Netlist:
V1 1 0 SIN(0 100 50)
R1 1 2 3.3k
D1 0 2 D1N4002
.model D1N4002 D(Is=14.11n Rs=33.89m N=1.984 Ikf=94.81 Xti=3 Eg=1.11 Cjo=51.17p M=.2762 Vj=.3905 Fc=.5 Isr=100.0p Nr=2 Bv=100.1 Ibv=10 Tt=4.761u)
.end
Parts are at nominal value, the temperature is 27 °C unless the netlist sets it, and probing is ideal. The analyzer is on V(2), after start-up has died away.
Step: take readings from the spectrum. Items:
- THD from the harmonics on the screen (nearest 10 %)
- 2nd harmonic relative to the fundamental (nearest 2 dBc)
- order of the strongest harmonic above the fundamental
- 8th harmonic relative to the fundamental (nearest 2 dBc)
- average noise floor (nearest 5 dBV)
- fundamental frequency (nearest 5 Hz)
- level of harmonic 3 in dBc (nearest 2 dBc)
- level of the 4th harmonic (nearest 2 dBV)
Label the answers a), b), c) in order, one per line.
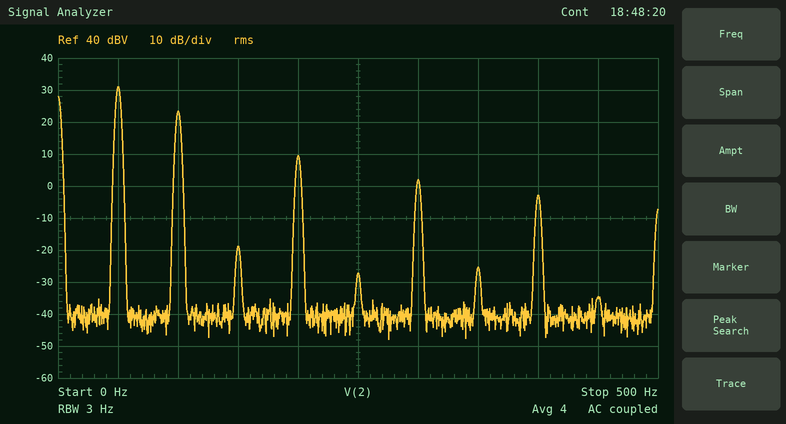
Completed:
a) 40 %
b) -8 dBc
c) 2
d) -34 dBc
e) -40 dBV
f) 50 Hz
g) -50 dBc
h) 10 dBV
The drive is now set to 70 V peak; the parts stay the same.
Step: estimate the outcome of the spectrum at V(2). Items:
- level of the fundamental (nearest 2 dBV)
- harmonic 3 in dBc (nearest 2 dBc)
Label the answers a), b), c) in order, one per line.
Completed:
a) 28 dBV
b) -48 dBc
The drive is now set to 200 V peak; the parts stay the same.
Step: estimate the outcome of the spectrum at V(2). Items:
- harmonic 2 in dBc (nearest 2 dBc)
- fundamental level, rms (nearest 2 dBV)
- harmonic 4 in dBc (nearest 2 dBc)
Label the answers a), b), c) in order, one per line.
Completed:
a) -12 dBc
b) 32 dBV
c) -14 dBc
